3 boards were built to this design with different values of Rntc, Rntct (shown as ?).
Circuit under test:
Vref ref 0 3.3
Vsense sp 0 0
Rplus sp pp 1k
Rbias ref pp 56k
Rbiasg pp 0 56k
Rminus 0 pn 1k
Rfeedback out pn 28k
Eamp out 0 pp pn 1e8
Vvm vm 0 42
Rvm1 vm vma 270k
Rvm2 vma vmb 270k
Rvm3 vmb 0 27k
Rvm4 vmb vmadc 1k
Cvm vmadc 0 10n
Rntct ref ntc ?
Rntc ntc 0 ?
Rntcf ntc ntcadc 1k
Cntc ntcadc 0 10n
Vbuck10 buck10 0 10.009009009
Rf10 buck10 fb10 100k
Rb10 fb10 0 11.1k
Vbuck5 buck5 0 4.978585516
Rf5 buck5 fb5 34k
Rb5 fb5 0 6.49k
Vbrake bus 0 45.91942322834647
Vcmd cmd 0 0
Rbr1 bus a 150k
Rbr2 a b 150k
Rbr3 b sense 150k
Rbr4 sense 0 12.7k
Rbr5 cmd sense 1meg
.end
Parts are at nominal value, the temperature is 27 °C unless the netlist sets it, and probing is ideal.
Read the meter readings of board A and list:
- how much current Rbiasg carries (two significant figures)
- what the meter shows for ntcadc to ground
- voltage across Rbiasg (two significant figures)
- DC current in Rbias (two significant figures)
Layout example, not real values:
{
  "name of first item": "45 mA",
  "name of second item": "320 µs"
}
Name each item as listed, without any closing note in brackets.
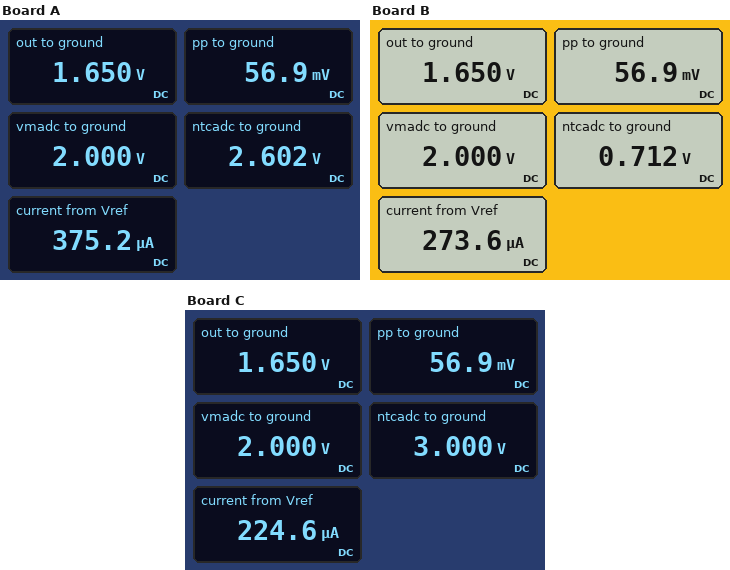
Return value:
{
  "how much current Rbiasg carries": "1.0 µA",
  "what the meter shows for ntcadc to ground": "2.602 V",
  "voltage across Rbiasg": "57 mV",
  "DC current in Rbias": "58 µA"
}
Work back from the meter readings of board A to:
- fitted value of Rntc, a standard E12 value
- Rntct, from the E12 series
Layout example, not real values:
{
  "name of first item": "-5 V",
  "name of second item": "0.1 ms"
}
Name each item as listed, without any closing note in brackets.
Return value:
{
  "fitted value of Rntc, a standard E12 value": "8.2 kΩ",
  "Rntct, from the E12 series": "2.2 kΩ"
}
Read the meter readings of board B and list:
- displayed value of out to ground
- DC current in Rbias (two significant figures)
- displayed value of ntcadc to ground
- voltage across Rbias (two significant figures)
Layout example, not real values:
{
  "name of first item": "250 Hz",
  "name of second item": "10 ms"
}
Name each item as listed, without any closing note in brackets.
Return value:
{
  "displayed value of out to ground": "1.650 V",
  "DC current in Rbias": "58 µA",
  "displayed value of ntcadc to ground": "0.712 V",
  "voltage across Rbias": "3.2 V"
}
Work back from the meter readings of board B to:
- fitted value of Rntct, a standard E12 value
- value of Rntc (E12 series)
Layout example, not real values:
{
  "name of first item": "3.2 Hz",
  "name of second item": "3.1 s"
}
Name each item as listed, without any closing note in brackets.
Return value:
{
  "fitted value of Rntct, a standard E12 value": "12 kΩ",
  "value of Rntc": "3.3 kΩ"
}
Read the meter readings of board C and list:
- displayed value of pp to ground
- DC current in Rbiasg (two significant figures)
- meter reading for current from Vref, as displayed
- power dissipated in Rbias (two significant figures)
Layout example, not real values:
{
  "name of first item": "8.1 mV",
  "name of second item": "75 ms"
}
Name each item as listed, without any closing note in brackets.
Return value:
{
  "displayed value of pp to ground": "56.9 mV",
  "DC current in Rbiasg": "1.0 µA",
  "meter reading for current from Vref, as displayed": "224.6 µA",
  "power dissipated in Rbias": "190 µW"
}
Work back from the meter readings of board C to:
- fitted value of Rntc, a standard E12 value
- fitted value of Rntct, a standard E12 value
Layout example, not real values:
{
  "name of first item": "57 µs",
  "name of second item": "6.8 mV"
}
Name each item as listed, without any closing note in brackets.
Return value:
{
  "fitted value of Rntc, a standard E12 value": "18 kΩ",
  "fitted value of Rntct, a standard E12 value": "1.8 kΩ"
}
